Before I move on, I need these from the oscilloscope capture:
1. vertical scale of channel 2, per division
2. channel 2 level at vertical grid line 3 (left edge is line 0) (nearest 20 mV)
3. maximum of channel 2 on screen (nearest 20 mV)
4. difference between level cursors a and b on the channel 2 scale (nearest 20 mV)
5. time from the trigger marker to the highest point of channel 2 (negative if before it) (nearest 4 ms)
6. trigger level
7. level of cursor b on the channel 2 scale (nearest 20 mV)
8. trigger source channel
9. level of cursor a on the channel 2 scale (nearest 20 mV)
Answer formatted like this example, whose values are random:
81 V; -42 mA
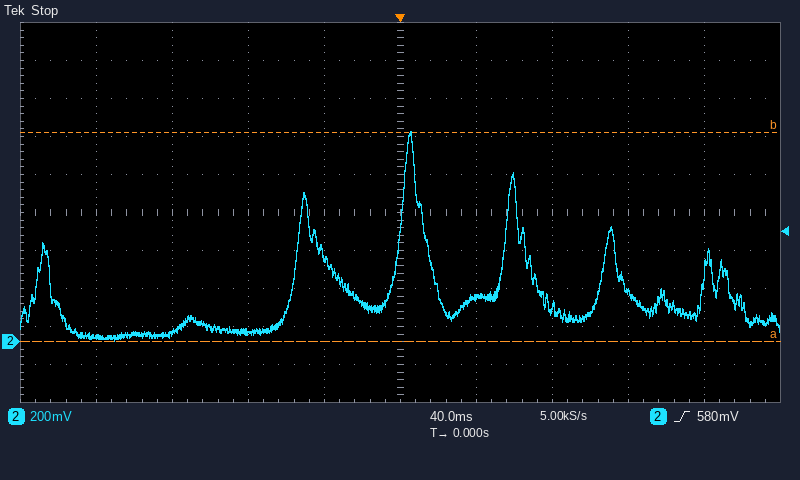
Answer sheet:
200 mV; 60 mV; 1.10 V; 1.10 V; +4 ms; 580 mV; 1.10 V; channel 2; 0 mV
